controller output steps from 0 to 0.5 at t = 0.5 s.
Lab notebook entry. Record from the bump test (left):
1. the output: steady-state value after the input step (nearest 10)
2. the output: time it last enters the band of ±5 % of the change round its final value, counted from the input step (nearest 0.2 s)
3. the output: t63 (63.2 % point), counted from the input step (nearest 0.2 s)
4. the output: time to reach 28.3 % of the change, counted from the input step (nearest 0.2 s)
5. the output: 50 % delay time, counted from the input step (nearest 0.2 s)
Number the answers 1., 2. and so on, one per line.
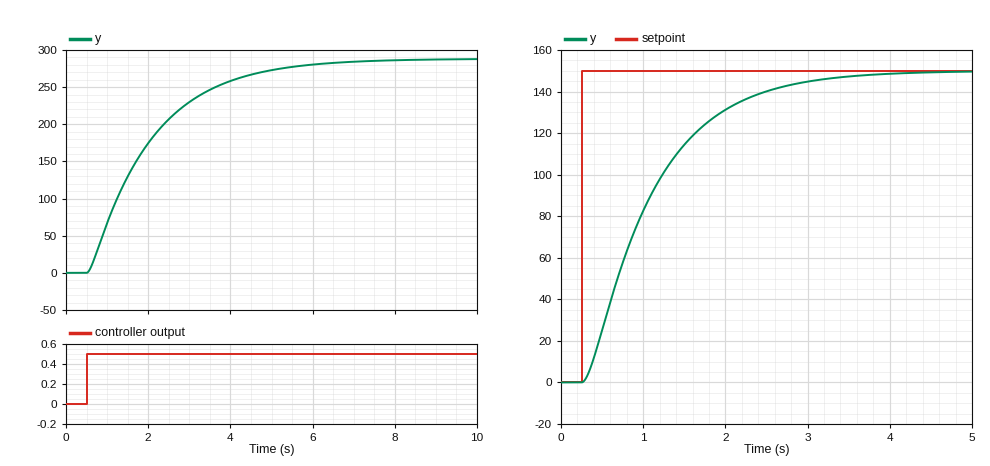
1. 290
2. 4.6 s
3. 1.6 s
4. 0.6 s
5. 1.2 s
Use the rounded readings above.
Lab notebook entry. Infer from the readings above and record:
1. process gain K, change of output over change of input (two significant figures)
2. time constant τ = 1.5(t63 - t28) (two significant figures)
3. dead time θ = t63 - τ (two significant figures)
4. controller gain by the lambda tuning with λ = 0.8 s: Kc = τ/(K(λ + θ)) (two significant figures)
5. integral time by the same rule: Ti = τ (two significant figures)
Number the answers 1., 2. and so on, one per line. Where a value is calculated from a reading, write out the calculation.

1. (290 - 0) / 0.5 = 580
2. 1.5 × (1.6 - 0.6) = 1.5 s
3. 1.6 - 1.5 = 0.10 s
4. 1.5 / (580 × (0.8 + 0.1)) = 0.0029
5. 1.5 s
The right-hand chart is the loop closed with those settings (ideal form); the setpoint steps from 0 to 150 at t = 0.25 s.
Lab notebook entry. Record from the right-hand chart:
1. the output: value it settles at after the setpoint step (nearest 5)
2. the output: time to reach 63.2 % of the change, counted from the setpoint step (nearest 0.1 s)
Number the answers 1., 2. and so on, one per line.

1. 150
2. 0.9 s
